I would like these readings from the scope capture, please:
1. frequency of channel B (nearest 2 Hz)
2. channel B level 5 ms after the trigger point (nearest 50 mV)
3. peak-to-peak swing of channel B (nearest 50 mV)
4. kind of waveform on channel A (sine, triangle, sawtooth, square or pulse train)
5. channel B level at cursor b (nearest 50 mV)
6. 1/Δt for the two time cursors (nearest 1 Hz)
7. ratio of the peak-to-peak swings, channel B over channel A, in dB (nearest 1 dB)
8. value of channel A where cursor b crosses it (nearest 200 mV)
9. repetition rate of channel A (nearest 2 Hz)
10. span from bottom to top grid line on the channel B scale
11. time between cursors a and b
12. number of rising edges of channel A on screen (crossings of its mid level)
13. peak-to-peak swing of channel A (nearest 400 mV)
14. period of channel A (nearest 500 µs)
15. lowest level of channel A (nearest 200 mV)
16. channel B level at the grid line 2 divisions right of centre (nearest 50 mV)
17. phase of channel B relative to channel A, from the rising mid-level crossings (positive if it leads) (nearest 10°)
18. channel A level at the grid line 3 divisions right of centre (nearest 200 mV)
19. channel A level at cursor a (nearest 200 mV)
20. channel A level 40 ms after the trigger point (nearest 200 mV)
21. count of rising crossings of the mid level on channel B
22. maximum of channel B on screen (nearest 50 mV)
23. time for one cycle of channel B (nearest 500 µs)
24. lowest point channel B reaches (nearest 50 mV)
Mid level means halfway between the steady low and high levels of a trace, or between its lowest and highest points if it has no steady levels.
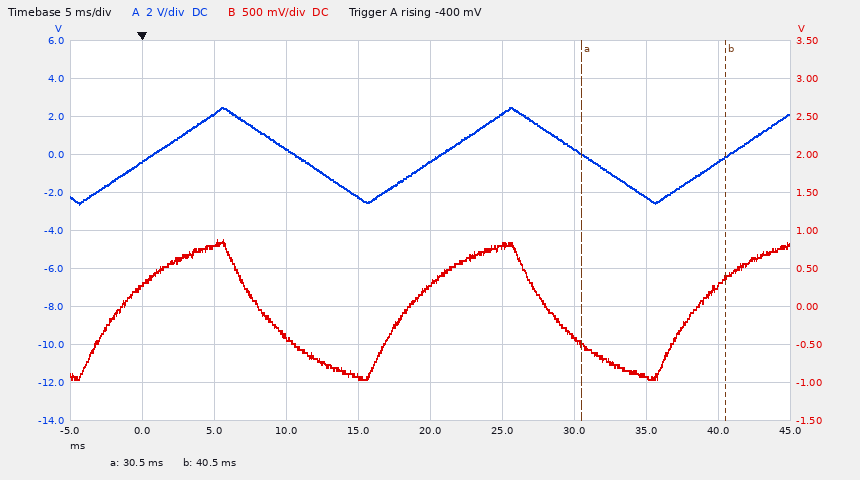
50 Hz
800 mV
1.85 V
triangle
350 mV
100 Hz
-9 dB
-200 mV
50 Hz
5 V
10.0 ms
3
5.2 V
20.0 ms
-2.6 V
-400 mV
+40°
-2.2 V
0.0 V
-400 mV
3
900 mV
20.0 ms
-950 mV
